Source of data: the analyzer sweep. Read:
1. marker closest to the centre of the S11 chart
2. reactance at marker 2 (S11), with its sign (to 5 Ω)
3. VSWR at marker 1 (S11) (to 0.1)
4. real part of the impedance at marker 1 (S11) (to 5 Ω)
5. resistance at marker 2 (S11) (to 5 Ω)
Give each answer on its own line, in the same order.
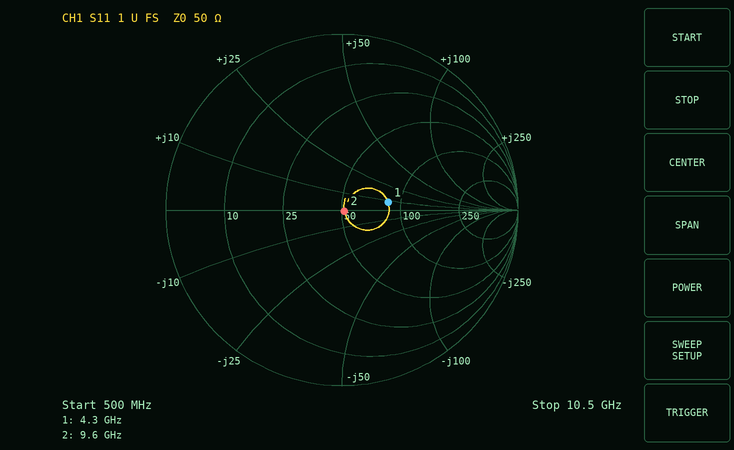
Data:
marker 2
0 Ω
1.7
85 Ω
50 Ω
